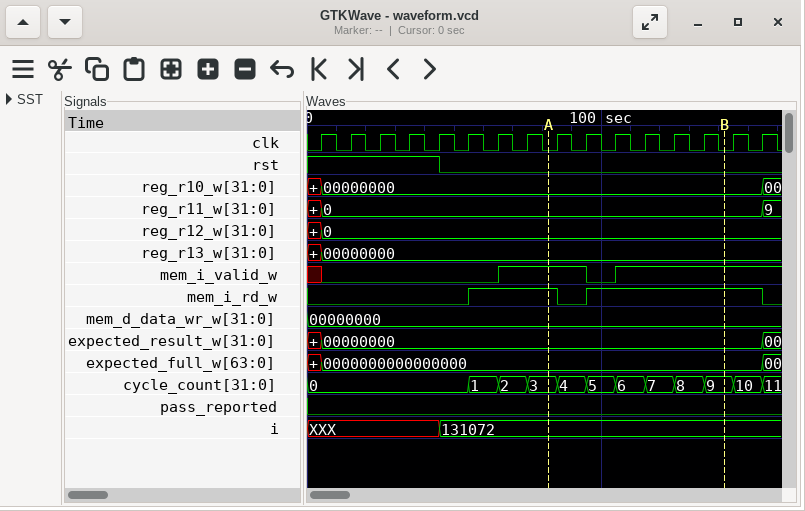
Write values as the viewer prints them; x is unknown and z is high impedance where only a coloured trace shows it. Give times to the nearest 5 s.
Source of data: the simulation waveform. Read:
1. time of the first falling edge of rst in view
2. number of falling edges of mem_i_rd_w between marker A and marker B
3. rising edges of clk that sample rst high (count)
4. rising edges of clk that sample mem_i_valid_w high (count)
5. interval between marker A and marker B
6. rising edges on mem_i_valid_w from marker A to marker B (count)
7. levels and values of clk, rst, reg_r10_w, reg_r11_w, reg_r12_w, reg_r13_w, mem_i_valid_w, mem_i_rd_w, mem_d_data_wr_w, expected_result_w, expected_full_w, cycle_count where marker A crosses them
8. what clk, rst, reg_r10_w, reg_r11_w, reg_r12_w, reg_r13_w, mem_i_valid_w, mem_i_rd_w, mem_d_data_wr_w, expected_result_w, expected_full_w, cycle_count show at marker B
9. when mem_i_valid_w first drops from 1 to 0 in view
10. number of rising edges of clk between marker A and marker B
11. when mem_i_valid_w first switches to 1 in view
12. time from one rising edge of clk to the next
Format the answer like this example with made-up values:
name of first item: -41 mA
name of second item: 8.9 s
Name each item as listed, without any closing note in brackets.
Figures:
time of the first falling edge of rst in view: 45 s
number of falling edges of mem_i_rd_w between marker A and marker B: 1
rising edges of clk that sample rst high: 5
rising edges of clk that sample mem_i_valid_w high: 8
interval between marker A and marker B: 60 s
rising edges on mem_i_valid_w from marker A to marker B: 1
levels and values of clk, rst, reg_r10_w, reg_r11_w, reg_r12_w, reg_r13_w, mem_i_valid_w, mem_i_rd_w, mem_d_data_wr_w, expected_result_w, expected_full_w, cycle_count where marker A crosses them: clk=0, rst=0, reg_r10_w=00000000, reg_r11_w=0, reg_r12_w=0, reg_r13_w=00000000, mem_i_valid_w=1, mem_i_rd_w=1, mem_d_data_wr_w=00000000, expected_result_w=00000000, expected_full_w=0000000000000000, cycle_count=3
what clk, rst, reg_r10_w, reg_r11_w, reg_r12_w, reg_r13_w, mem_i_valid_w, mem_i_rd_w, mem_d_data_wr_w, expected_result_w, expected_full_w, cycle_count show at marker B: clk=0, rst=0, reg_r10_w=00000000, reg_r11_w=0, reg_r12_w=0, reg_r13_w=00000000, mem_i_valid_w=1, mem_i_rd_w=1, mem_d_data_wr_w=00000000, expected_result_w=00000000, expected_full_w=0000000000000000, cycle_count=9
when mem_i_valid_w first drops from 1 to 0 in view: 95 s
number of rising edges of clk between marker A and marker B: 6
when mem_i_valid_w first switches to 1 in view: 65 s
time from one rising edge of clk to the next: 10 s
